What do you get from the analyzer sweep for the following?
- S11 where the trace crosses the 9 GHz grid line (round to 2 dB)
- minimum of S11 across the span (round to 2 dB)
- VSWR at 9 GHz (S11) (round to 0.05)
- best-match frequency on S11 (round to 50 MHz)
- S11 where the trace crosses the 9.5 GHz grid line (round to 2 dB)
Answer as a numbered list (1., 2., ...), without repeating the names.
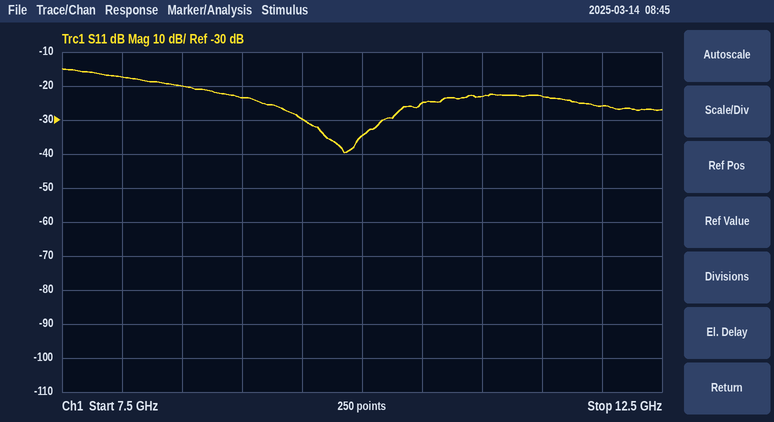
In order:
1. -24 dB
2. -40 dB
3. 1.15
4. 9.85 GHz
5. -30 dB
